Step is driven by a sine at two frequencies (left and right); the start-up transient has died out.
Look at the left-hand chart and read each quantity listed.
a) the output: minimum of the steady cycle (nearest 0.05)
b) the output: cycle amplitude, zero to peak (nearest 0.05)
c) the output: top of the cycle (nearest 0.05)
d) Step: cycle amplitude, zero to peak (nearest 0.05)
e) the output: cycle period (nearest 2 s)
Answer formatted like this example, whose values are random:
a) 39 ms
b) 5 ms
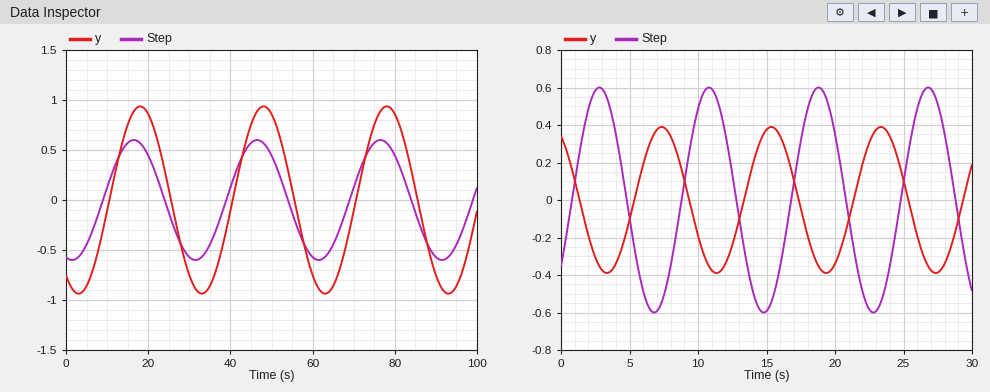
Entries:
a) -0.95
b) 0.95
c) 0.95
d) 0.60
e) 30 s
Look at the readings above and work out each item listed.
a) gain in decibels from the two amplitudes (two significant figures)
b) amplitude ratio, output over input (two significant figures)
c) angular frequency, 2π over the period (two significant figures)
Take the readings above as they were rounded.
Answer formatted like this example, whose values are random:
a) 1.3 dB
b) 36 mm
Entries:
a) 4.0 dB
b) 1.6
c) 0.21 rad/s
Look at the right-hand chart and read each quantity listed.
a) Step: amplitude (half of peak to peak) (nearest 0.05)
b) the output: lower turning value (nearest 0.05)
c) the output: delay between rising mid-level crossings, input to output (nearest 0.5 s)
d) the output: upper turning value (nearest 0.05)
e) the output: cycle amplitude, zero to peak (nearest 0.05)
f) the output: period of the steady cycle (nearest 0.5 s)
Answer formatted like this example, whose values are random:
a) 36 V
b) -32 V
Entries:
a) 0.60
b) -0.40
c) 4.5 s
d) 0.40
e) 0.40
f) 8.0 s
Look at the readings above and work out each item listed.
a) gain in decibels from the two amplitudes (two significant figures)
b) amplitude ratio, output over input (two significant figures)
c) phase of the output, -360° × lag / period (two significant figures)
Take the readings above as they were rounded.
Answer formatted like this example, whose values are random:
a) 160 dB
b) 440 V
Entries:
a) -3.5 dB
b) 0.67
c) -200°
